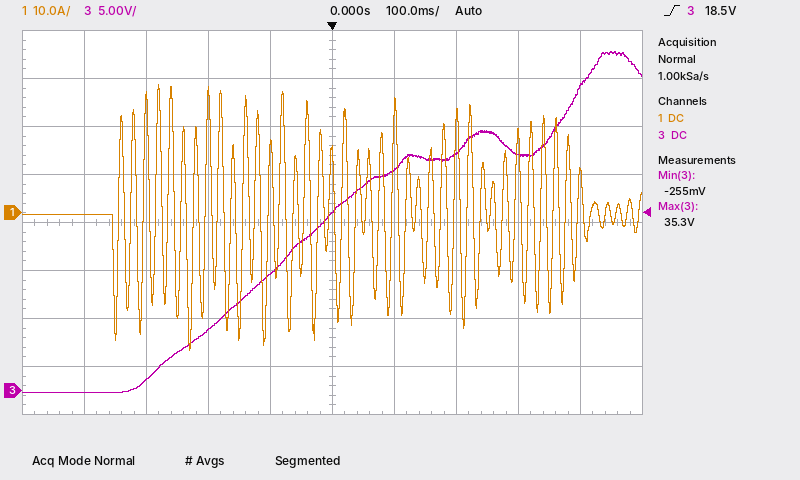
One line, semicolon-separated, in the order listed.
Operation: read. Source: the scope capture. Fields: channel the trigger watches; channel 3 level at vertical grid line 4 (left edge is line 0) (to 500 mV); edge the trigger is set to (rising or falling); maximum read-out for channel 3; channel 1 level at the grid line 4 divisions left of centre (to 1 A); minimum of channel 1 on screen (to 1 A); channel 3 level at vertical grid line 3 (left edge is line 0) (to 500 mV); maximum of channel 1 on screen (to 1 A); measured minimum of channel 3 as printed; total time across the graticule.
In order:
channel 3; 12.0 V; rising; 35.3 V; 0 A; -29 A; 6.5 V; 27 A; -255 mV; 1 s
